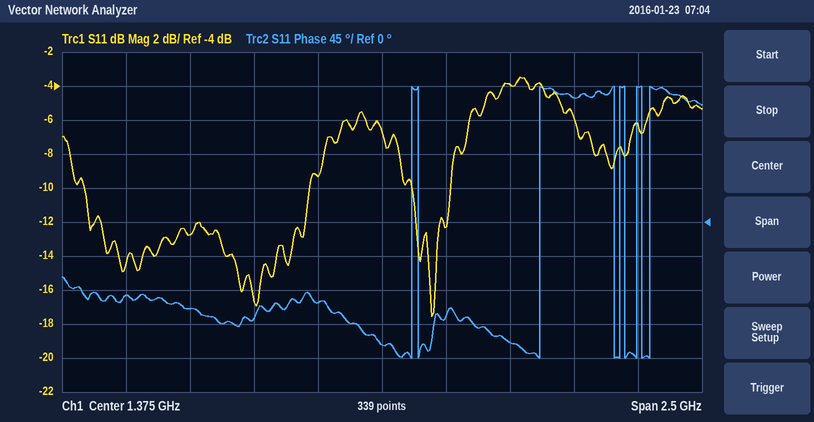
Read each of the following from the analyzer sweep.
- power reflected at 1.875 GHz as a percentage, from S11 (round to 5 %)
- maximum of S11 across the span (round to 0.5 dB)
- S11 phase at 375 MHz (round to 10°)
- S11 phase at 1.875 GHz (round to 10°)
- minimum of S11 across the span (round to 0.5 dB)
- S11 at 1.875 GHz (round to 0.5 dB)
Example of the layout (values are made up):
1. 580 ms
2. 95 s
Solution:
1. 40 %
2. -3.5 dB
3. -100°
4. -160°
5. -17.5 dB
6. -4.0 dB
